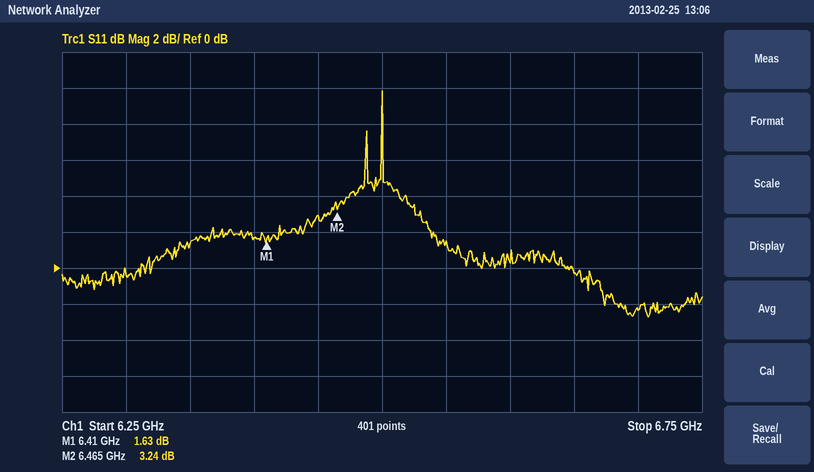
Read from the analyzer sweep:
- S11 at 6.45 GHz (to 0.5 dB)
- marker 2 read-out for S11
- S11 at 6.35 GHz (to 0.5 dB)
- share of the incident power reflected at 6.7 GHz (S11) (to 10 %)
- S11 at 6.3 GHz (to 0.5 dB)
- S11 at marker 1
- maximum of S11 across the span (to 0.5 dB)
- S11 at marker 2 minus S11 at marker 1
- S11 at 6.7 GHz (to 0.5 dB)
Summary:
3.0 dB
3.24 dB
1.5 dB
60 %
-0.5 dB
1.63 dB
10.0 dB
1.61 dB
-2.5 dB
